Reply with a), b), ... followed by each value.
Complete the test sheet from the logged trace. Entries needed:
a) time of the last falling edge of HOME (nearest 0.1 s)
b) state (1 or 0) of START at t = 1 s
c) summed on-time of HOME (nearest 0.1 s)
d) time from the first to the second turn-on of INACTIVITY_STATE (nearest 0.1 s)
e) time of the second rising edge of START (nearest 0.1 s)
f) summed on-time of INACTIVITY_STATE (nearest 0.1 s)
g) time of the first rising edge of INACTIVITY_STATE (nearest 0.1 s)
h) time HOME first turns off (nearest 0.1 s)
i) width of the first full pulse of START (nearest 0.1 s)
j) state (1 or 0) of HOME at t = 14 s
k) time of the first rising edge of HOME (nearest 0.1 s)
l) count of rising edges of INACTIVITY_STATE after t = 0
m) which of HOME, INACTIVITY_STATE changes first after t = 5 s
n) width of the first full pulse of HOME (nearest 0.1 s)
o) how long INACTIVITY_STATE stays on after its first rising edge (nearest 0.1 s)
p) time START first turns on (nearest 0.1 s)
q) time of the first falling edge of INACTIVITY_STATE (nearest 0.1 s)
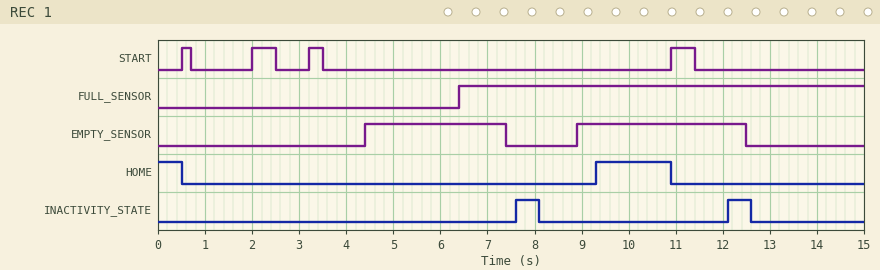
a) 10.9 s
b) 0
c) 2.1 s
d) 4.5 s
e) 2.0 s
f) 1.0 s
g) 7.6 s
h) 0.5 s
i) 0.2 s
j) 0
k) 9.3 s
l) 2
m) INACTIVITY_STATE
n) 1.6 s
o) 0.5 s
p) 0.5 s
q) 8.1 s
